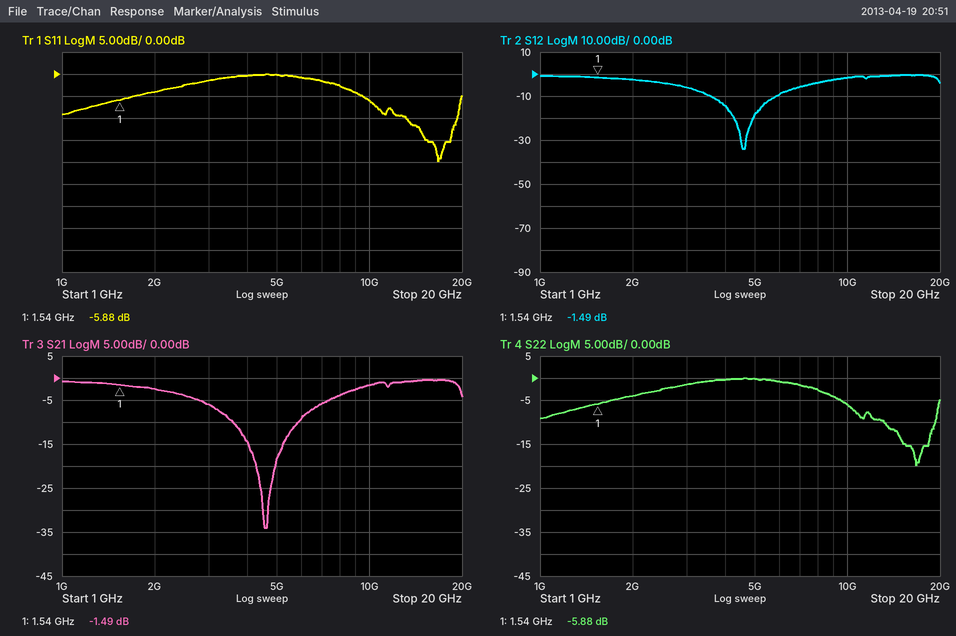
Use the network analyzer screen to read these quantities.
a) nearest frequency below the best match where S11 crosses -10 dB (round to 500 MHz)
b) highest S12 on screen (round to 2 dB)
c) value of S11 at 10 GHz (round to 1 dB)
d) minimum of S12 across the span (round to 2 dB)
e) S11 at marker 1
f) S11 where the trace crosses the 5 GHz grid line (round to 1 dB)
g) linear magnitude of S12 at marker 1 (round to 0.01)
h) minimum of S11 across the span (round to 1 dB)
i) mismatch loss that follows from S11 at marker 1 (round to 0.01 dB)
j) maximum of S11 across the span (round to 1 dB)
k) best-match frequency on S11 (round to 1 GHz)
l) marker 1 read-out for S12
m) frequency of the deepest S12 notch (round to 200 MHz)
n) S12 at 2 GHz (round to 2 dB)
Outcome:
13.0 GHz
0 dB
-6 dB
-34 dB
-5.88 dB
0 dB
0.84
-20 dB
1.30 dB
0 dB
17 GHz
-1.49 dB
4.6 GHz
-2 dB
